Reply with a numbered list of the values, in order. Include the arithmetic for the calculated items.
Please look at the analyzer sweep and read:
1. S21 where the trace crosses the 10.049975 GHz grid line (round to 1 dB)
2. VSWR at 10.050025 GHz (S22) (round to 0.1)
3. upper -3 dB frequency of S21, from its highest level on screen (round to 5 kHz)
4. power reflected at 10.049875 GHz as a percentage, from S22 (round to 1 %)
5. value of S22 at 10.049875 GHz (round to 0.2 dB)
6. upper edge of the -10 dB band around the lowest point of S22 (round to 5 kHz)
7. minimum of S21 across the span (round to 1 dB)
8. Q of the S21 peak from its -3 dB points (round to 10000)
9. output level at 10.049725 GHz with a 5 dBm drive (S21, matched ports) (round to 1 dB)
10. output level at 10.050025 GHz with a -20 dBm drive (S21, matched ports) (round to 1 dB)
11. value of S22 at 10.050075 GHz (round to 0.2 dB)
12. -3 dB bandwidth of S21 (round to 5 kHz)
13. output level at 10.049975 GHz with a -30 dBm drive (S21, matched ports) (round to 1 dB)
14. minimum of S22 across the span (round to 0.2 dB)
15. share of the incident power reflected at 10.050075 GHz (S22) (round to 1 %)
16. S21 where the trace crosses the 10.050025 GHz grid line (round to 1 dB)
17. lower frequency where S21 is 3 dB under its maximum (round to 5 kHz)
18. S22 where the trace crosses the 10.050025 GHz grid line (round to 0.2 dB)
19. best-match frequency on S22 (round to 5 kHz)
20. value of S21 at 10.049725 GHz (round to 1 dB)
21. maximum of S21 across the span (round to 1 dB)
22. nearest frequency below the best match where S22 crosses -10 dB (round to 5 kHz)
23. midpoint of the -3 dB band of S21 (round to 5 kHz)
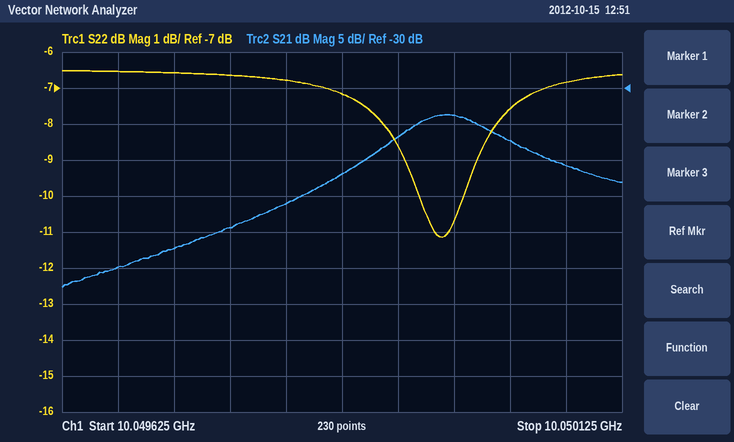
1. -34 dB
2. |Γ| = 10^(-7.6/20) = 0.4169; VSWR = (1 + 0.4169)/(1 − 0.4169) ≈ 2.4
3. 10.050015 GHz
4. 10^(-7.2/10) ≈ 19 %
5. -7.2 dB
6. 10.049985 GHz
7. -58 dB
8. 10.05 GHz / 90 kHz ≈ 111666, so 110000 to the nearest 10000
9. 5 dBm + (-52 dB) = -47 dBm
10. -20 dBm + (-37 dB) = -57 dBm
11. -6.8 dB
12. 10.050015 GHz − 10.049925 GHz = 90 kHz
13. -30 dBm + (-34 dB) = -64 dBm
14. -11.2 dB
15. 10^(-6.8/10) ≈ 21 %
16. -37 dB
17. 10.049925 GHz
18. -7.6 dB
19. 10.049965 GHz
20. -52 dB
21. -34 dB
22. 10.049945 GHz
23. 10.049970 GHz
